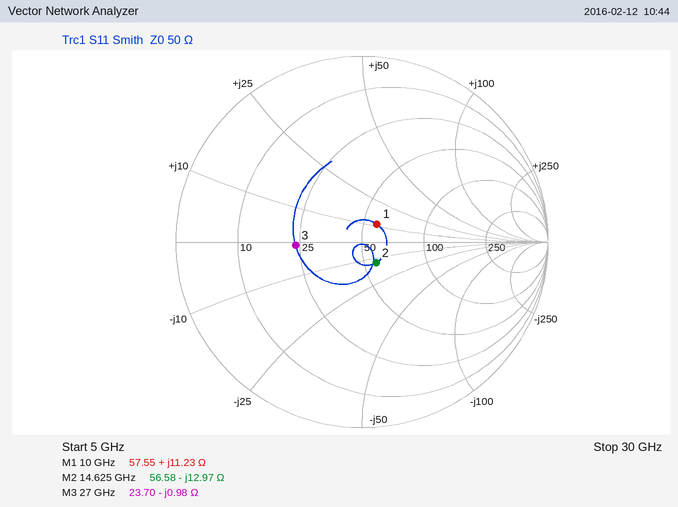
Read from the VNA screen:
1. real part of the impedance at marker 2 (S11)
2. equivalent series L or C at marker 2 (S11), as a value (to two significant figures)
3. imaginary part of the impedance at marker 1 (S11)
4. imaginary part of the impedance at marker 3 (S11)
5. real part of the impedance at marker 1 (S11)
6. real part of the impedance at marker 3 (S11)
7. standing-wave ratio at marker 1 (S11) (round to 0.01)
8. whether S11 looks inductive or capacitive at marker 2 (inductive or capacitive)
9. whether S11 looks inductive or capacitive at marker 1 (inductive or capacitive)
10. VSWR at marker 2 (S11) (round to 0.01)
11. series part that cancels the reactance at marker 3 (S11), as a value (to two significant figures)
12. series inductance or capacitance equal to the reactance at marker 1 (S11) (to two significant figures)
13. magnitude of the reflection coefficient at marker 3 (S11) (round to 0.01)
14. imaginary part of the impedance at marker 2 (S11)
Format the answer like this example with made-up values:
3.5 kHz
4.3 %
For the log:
56.58 Ω
840 fF
+11.23 Ω
-0.98 Ω
57.55 Ω
23.70 Ω
1.29
capacitive
inductive
1.31
5.8 pH
180 pH
0.36
-12.97 Ω
